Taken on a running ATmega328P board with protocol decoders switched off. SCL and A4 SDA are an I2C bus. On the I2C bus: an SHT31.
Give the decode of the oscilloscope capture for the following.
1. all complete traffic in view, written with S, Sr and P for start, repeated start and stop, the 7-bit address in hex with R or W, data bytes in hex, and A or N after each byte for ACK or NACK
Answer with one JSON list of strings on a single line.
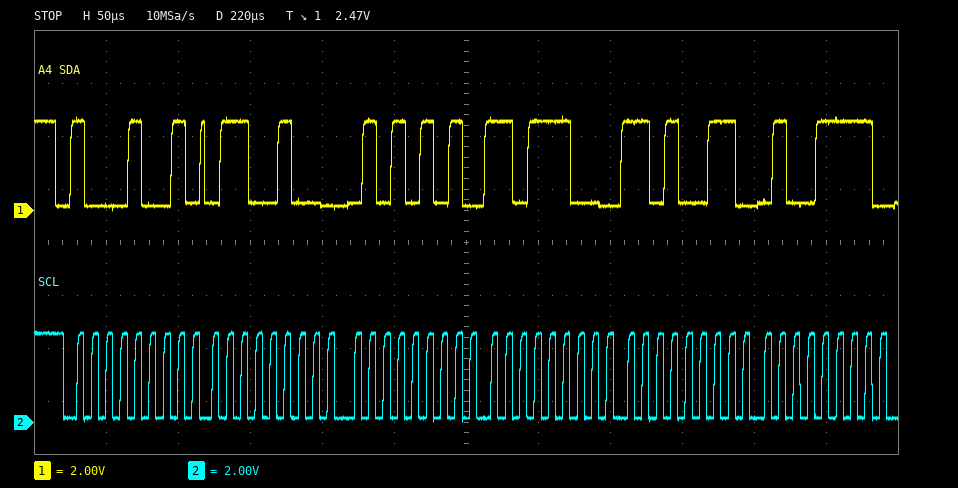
["S 44R A 64 A 55 A DC A D3 A 4F A"]
